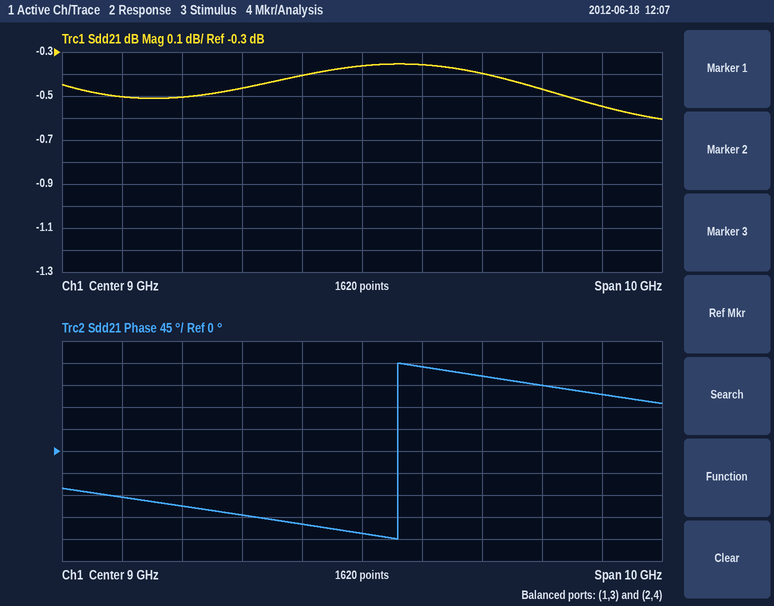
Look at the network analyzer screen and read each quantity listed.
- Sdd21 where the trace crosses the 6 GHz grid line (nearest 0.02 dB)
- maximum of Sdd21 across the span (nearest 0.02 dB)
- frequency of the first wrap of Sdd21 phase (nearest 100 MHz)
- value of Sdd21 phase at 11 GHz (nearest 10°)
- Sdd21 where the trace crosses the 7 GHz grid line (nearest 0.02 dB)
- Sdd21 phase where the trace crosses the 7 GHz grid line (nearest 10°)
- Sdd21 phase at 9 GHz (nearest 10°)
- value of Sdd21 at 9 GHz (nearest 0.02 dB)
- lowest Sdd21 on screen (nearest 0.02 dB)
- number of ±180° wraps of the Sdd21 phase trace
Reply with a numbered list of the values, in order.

1. -0.50 dB
2. -0.36 dB
3. 9.6 GHz
4. 150°
5. -0.46 dB
6. -130°
7. -170°
8. -0.36 dB
9. -0.60 dB
10. 1
